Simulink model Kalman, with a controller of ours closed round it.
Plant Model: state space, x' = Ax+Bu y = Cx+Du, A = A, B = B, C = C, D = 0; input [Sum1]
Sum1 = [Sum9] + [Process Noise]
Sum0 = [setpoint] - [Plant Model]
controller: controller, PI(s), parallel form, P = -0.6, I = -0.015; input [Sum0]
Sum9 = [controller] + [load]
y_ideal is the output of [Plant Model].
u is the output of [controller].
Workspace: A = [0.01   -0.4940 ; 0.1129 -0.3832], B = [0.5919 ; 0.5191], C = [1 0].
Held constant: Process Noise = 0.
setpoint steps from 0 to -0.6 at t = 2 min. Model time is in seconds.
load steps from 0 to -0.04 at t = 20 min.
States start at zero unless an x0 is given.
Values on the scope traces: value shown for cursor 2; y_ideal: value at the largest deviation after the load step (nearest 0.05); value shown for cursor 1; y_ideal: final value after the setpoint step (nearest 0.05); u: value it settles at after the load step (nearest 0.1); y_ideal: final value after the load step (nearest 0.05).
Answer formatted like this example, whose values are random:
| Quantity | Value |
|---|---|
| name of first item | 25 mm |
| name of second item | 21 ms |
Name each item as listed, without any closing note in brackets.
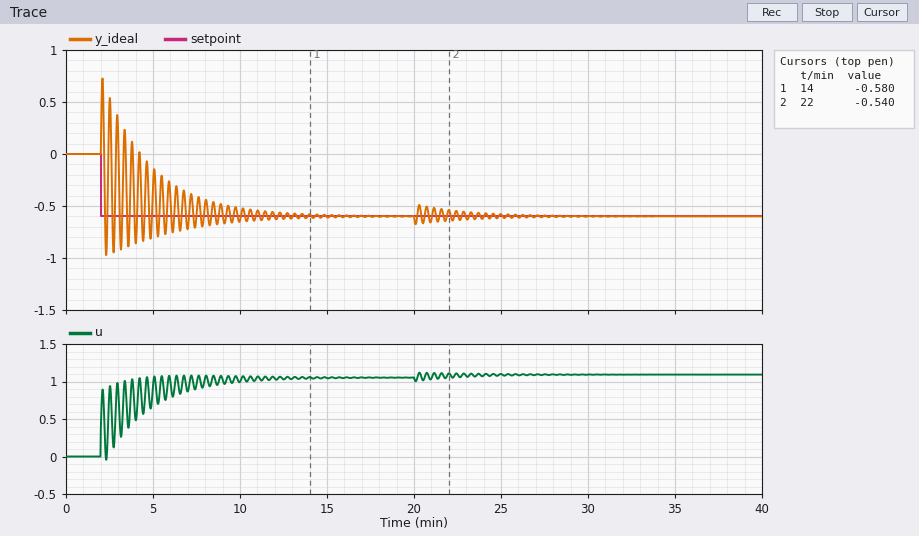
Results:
| Quantity | Value |
|---|---|
| value shown for cursor 2 | -0.540 |
| y_ideal: value at the largest deviation after the load step | -0.50 |
| value shown for cursor 1 | -0.580 |
| y_ideal: final value after the setpoint step | -0.60 |
| u: value it settles at after the load step | 1.1 |
| y_ideal: final value after the load step | -0.60 |
